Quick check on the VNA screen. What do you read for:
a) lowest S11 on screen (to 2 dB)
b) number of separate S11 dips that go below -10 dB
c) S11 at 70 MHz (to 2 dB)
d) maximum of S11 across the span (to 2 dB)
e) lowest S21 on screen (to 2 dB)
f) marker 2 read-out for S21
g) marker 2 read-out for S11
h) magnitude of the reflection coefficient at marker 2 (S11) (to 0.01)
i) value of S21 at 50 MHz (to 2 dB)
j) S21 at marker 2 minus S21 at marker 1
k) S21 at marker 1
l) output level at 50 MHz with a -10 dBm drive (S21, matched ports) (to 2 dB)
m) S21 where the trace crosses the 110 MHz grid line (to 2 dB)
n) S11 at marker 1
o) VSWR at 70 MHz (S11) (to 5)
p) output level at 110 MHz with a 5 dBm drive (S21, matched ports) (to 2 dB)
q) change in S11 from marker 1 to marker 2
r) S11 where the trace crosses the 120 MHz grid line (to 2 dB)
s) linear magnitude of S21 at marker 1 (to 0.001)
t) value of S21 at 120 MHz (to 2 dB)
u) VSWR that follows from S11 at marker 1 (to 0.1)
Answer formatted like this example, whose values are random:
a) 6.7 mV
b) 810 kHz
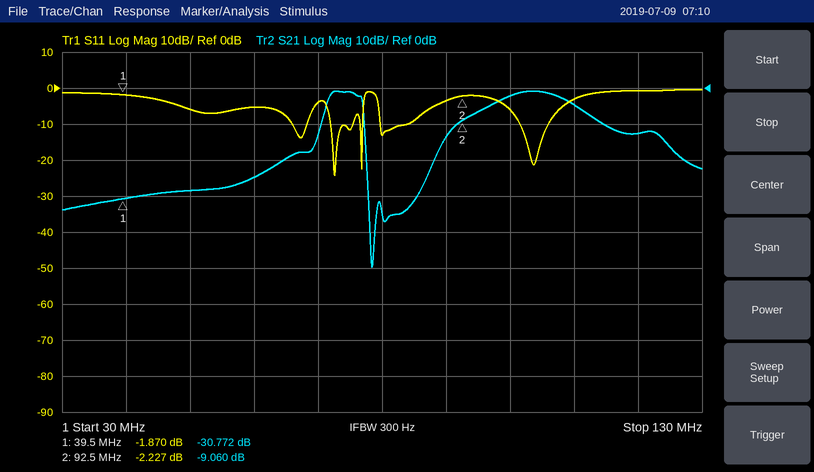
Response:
a) -24 dB
b) 5
c) -4 dB
d) 0 dB
e) -50 dB
f) -9.060 dB
g) -2.227 dB
h) 0.77
i) -28 dB
j) 21.712 dB
k) -30.772 dB
l) -38 dBm
m) -4 dB
n) -1.870 dB
o) 5
p) 0 dBm
q) -0.357 dB
r) 0 dB
s) 0.029
t) -12 dB
u) 9.3
